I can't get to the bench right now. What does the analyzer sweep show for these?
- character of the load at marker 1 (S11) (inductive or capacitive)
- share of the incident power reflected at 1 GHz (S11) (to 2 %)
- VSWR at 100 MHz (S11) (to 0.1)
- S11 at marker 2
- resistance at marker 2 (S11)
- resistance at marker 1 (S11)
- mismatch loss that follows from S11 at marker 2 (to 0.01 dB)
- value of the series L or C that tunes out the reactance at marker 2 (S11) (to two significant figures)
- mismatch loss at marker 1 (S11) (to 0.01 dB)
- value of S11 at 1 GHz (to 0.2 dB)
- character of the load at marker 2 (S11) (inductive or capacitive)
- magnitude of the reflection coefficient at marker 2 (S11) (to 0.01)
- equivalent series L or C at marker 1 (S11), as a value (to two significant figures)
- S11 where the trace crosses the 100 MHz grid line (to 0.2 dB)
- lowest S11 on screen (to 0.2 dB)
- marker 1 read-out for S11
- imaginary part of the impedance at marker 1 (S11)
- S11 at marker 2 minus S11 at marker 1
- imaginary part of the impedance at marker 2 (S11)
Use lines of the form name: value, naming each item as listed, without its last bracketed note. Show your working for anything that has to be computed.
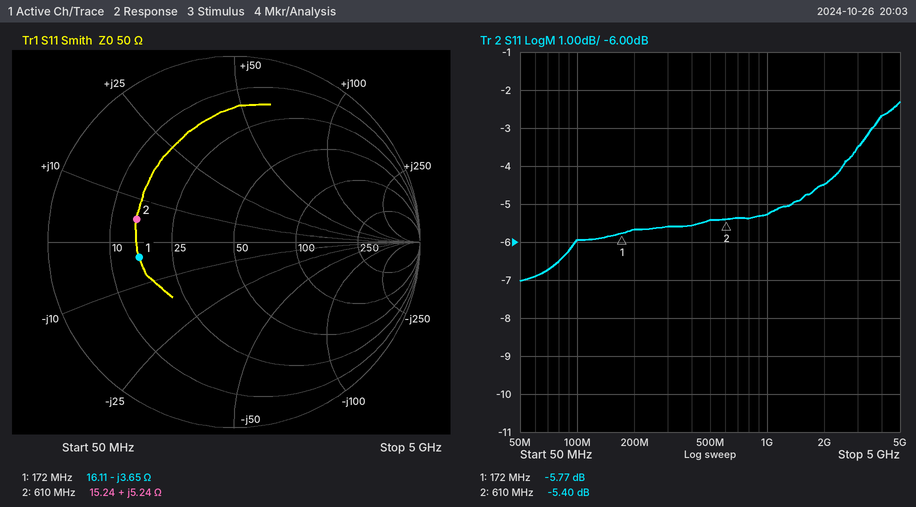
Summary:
character of the load at marker 1 (S11): capacitive
share of the incident power reflected at 1 GHz (S11): 10^(-5.2/10) ≈ 30 %
VSWR at 100 MHz (S11): |Γ| = 10^(-6/20) = 0.5012; VSWR = (1 + 0.5012)/(1 − 0.5012) ≈ 3.0
S11 at marker 2: -5.40 dB
resistance at marker 2: 15.24 Ω
resistance at marker 1: 16.11 Ω
mismatch loss that follows from S11 at marker 2: −10 log10(1 − 10^(-5.4/10)) ≈ 1.48 dB
value of the series L or C that tunes out the reactance at marker 2 (S11): C = 1/(2π × 610 MHz × 5.24 Ω) ≈ 50 pF
mismatch loss at marker 1 (S11): −10 log10(1 − 10^(-5.77/10)) ≈ 1.34 dB
value of S11 at 1 GHz: -5.2 dB
character of the load at marker 2 (S11): inductive
magnitude of the reflection coefficient at marker 2 (S11): 0.54
equivalent series L or C at marker 1 (S11), as a value: C = 1/(2π × 172 MHz × 3.65 Ω) ≈ 254 pF, so 250 pF to two significant figures
S11 where the trace crosses the 100 MHz grid line: -6.0 dB
lowest S11 on screen: -7.0 dB
marker 1 read-out for S11: -5.77 dB
imaginary part of the impedance at marker 1: -3.65 Ω
S11 at marker 2 minus S11 at marker 1: -5.4 − (-5.77) = 0.37 dB
imaginary part of the impedance at marker 2: +5.24 Ω
